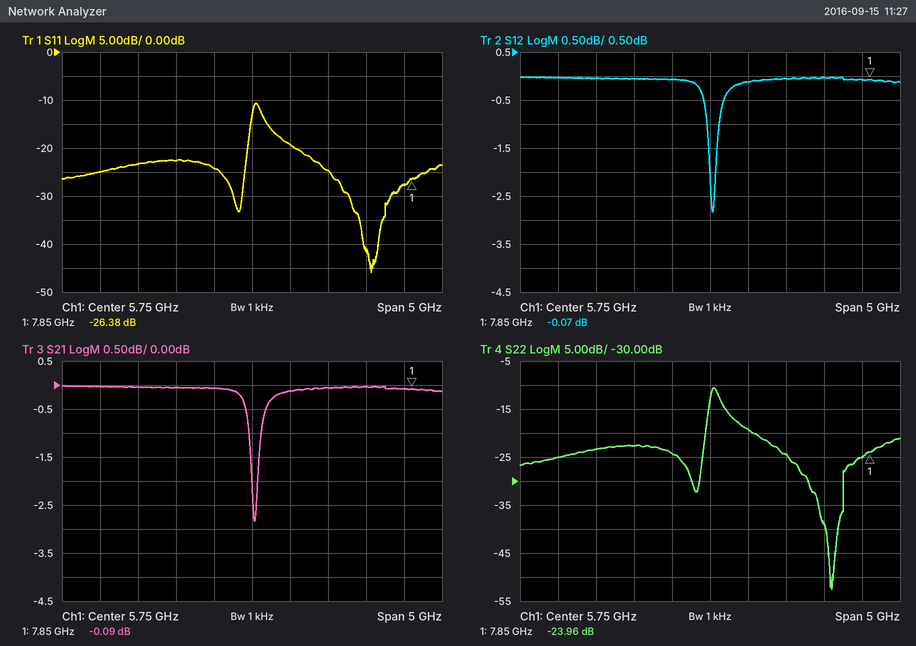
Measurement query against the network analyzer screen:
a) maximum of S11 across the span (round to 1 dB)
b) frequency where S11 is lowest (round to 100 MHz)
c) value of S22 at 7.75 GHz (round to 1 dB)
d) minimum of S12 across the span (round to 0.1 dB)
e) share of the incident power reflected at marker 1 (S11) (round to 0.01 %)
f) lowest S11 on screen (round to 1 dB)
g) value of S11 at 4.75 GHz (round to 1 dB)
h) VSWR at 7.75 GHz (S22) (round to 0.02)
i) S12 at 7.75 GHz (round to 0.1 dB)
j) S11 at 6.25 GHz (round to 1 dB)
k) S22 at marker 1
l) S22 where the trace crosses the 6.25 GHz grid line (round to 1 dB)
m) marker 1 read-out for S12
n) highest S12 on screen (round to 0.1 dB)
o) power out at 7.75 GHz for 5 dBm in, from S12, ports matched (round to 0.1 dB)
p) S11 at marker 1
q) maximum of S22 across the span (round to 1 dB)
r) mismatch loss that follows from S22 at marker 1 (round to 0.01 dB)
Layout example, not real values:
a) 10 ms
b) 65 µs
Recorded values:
a) -11 dB
b) 7.3 GHz
c) -25 dB
d) -2.8 dB
e) 0.23 %
f) -46 dB
g) -23 dB
h) 1.12
i) -0.1 dB
j) -19 dB
k) -23.96 dB
l) -19 dB
m) -0.07 dB
n) 0.0 dB
o) 4.9 dBm
p) -26.38 dB
q) -11 dB
r) 0.02 dB
